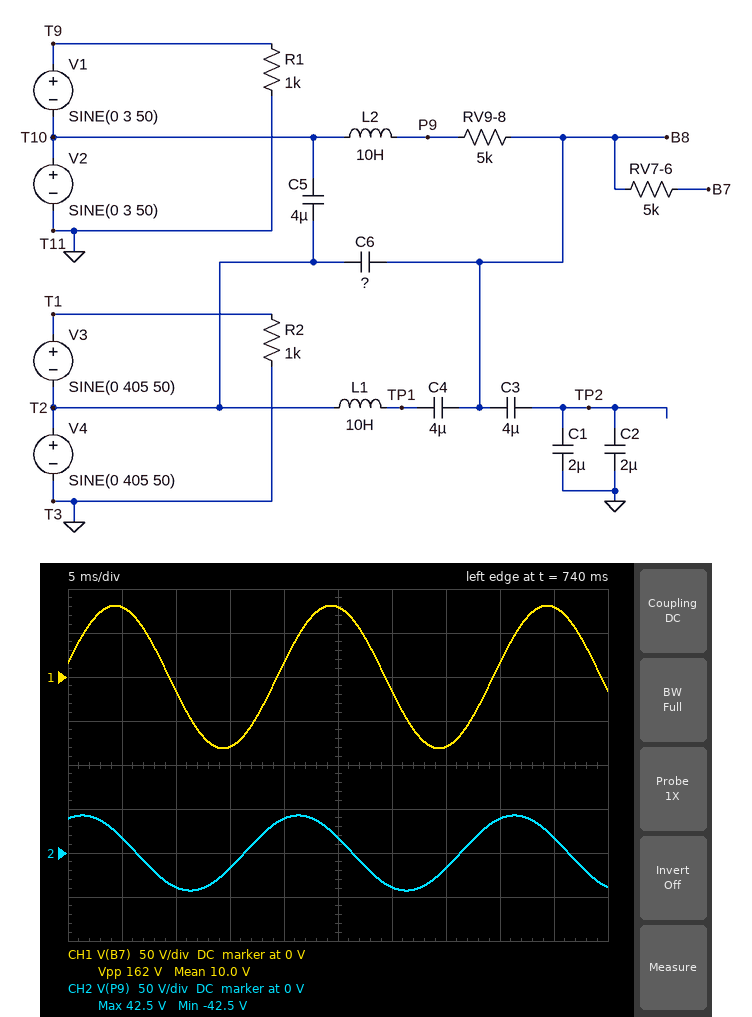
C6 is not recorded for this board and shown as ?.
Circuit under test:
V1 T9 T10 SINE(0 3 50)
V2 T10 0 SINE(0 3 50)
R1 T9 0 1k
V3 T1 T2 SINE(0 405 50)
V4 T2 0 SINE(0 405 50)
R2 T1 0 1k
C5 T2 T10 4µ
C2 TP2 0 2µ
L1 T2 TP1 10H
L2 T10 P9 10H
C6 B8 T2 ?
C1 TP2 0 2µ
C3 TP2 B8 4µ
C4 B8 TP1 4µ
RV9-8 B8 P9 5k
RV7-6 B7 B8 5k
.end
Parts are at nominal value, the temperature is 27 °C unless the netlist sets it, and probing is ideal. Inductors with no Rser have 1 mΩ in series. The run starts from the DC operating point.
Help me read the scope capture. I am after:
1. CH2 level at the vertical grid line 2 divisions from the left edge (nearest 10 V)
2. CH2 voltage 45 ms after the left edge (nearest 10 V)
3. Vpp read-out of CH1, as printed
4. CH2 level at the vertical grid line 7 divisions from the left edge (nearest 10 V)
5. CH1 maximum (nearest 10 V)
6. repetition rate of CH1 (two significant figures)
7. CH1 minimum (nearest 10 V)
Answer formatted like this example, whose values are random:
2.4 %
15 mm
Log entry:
-40 V
20 V
162 V
-20 V
80 V
50 Hz
-80 V
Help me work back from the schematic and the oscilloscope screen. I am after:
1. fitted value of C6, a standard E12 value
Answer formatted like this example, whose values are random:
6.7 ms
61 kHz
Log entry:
1.8 µF
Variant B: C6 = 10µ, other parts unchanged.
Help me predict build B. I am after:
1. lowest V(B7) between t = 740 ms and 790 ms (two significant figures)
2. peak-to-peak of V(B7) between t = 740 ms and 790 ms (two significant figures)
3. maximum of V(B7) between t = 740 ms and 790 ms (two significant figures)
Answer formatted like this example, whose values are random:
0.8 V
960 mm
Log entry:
-340 V
680 V
340 V
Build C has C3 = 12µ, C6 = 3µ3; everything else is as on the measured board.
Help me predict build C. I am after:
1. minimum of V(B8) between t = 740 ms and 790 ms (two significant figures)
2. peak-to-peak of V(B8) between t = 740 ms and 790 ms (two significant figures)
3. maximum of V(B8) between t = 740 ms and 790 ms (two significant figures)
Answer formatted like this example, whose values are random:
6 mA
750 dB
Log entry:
-170 V
340 V
170 V
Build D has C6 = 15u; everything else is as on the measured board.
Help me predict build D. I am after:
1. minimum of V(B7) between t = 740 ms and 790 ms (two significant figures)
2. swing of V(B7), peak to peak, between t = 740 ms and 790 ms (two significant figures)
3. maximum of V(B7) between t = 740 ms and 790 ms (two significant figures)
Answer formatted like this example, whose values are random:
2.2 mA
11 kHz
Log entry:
-360 V
720 V
360 V
